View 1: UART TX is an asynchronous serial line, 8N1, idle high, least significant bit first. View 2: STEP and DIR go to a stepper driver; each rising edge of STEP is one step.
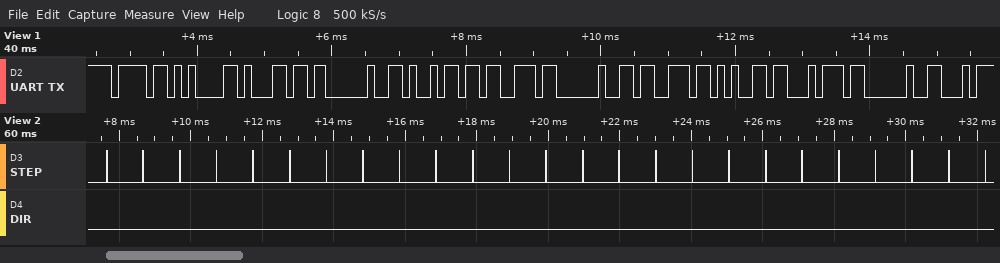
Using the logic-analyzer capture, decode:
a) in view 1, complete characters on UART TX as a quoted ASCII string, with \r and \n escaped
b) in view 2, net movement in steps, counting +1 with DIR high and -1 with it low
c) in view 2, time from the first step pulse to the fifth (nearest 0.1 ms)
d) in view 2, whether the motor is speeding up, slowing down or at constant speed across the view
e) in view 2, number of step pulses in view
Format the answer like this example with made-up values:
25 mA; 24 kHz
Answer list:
"oal is set "; -25; 4.1 ms; constant speed; 25
